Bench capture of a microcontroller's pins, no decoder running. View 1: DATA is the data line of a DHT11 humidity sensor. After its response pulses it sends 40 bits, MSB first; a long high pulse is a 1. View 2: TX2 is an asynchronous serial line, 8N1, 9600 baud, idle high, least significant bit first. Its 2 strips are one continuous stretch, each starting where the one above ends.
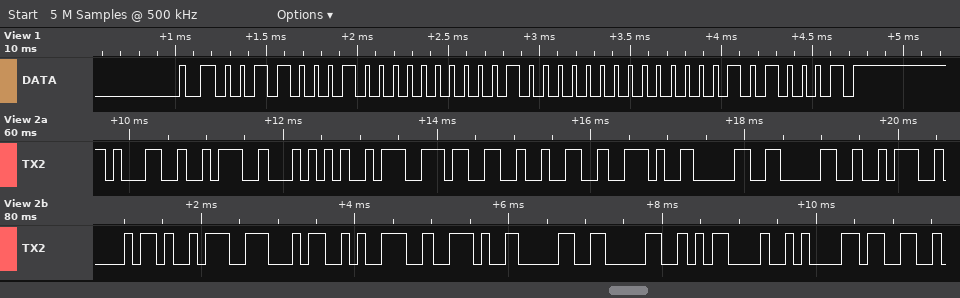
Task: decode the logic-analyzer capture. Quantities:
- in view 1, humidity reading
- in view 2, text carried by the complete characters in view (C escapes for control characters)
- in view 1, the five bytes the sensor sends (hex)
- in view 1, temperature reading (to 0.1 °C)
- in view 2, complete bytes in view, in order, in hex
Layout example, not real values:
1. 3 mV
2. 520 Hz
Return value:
1. 49 %
2. "1:T:32.00:h:49.00\r\n3"
3. 31 00 20 00 51
4. 32.0 °C
5. 31 3A 54 3A 33 32 2E 30 30 3A 68 3A 34 39 2E 30 30 0D 0A 33
